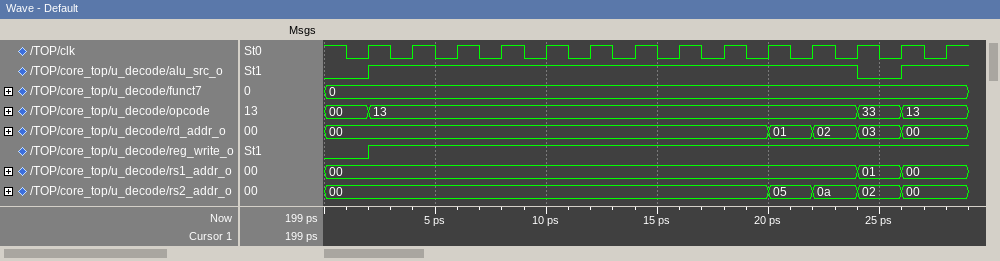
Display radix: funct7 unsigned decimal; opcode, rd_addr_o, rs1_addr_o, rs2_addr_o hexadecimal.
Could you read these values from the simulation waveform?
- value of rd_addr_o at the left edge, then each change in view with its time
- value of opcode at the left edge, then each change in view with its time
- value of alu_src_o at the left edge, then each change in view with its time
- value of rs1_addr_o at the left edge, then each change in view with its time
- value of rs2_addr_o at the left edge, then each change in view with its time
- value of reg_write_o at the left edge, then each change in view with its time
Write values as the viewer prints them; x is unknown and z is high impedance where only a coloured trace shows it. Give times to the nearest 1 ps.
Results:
00, 01 at 20 ps, 02 at 22 ps, 03 at 24 ps, 00 at 26 ps
00, 13 at 2 ps, 33 at 24 ps, 13 at 26 ps
0, 1 at 2 ps, 0 at 24 ps, 1 at 26 ps
00, 01 at 24 ps, 00 at 26 ps
00, 05 at 20 ps, 0a at 22 ps, 02 at 24 ps, 00 at 26 ps
0, 1 at 2 ps
